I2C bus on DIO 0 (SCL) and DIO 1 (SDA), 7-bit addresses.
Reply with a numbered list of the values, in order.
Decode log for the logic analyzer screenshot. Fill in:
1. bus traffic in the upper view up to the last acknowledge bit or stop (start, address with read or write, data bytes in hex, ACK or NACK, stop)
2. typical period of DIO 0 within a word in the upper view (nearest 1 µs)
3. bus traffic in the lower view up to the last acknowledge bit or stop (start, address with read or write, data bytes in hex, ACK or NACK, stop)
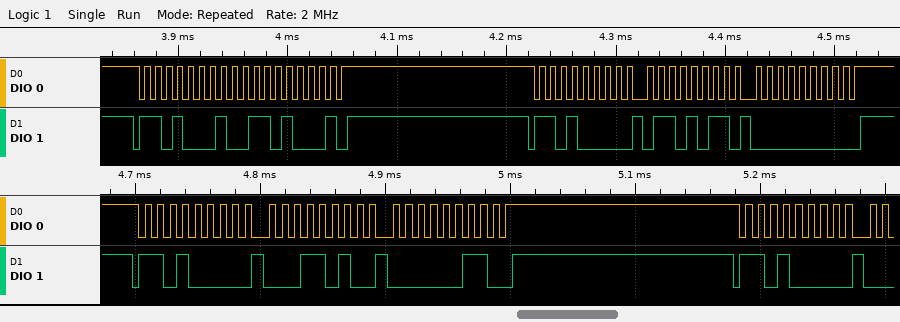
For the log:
1. start, address 68 read ACK, 68 NACK, stop, start, address 68 write ACK, 6B ACK, 00 ACK, stop
2. 10 µs
3. start, address 68 write ACK, 1A ACK, 03 ACK, stop, start, address 68 write ACK
